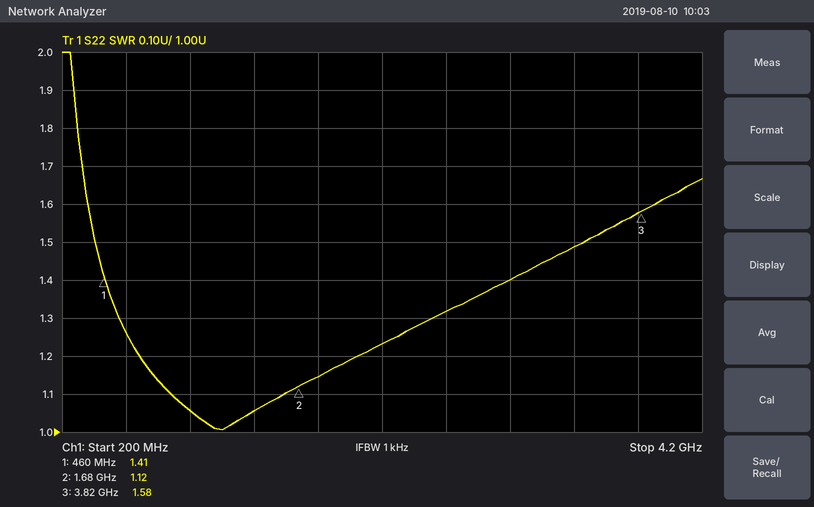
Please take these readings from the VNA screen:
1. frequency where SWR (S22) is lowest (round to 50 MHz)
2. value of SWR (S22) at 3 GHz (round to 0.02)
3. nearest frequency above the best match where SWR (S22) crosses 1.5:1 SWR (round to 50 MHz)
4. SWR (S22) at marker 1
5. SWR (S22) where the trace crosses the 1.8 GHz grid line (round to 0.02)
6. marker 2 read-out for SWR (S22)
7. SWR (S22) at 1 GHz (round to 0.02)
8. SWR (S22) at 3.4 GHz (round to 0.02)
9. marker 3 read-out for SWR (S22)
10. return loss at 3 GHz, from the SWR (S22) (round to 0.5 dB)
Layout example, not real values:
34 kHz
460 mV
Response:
1.20 GHz
1.40
3.45 GHz
1.41
1.14
1.12
1.06
1.48
1.58
15.5 dB
